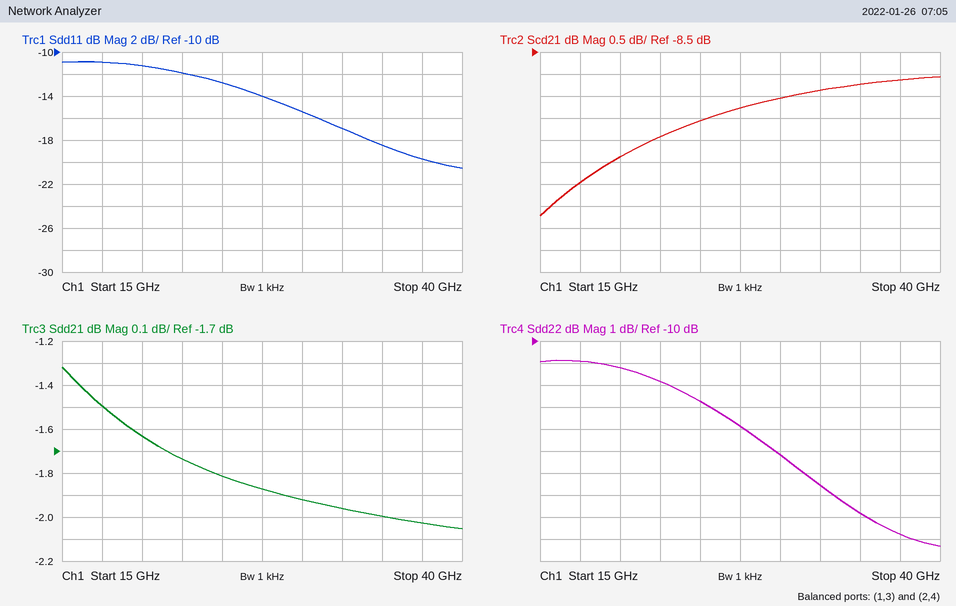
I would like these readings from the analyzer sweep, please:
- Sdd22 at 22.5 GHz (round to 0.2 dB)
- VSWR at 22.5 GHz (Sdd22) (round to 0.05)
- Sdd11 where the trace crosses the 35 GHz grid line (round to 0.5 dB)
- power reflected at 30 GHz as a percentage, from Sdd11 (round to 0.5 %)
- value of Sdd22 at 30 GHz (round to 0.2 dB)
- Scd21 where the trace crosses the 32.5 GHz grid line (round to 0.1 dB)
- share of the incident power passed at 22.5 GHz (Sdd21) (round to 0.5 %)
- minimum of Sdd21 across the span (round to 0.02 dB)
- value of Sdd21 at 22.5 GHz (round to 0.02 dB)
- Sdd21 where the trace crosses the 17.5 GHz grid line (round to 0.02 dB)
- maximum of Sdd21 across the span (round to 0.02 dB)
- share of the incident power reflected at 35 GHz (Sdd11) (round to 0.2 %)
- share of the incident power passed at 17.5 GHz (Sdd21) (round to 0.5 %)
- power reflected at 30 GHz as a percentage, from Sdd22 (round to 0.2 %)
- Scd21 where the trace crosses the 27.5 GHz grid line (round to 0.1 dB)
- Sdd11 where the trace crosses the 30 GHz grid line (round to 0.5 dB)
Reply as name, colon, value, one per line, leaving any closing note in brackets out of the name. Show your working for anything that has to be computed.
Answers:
Sdd22 at 22.5 GHz: -11.8 dB
VSWR at 22.5 GHz (Sdd22): |Γ| = 10^(-11.8/20) = 0.2570; VSWR = (1 + 0.2570)/(1 − 0.2570) ≈ 1.69, so 1.70 to the nearest 0.05
Sdd11 where the trace crosses the 35 GHz grid line: -18.5 dB
power reflected at 30 GHz as a percentage, from Sdd11: 10^(-15.5/10) ≈ 2.82 %, so 3.0 % to the nearest 0.5 %
value of Sdd22 at 30 GHz: -15.2 dB
Scd21 where the trace crosses the 32.5 GHz grid line: -9.4 dB
share of the incident power passed at 22.5 GHz (Sdd21): 10^(-1.74/10) ≈ 67.0 %
minimum of Sdd21 across the span: -2.06 dB
value of Sdd21 at 22.5 GHz: -1.74 dB
Sdd21 where the trace crosses the 17.5 GHz grid line: -1.50 dB
maximum of Sdd21 across the span: -1.32 dB
share of the incident power reflected at 35 GHz (Sdd11): 10^(-18.5/10) ≈ 1.4 %
share of the incident power passed at 17.5 GHz (Sdd21): 10^(-1.5/10) ≈ 70.8 %, so 71.0 % to the nearest 0.5 %
power reflected at 30 GHz as a percentage, from Sdd22: 10^(-15.2/10) ≈ 3.0 %
Scd21 where the trace crosses the 27.5 GHz grid line: -9.8 dB
Sdd11 where the trace crosses the 30 GHz grid line: -15.5 dB
